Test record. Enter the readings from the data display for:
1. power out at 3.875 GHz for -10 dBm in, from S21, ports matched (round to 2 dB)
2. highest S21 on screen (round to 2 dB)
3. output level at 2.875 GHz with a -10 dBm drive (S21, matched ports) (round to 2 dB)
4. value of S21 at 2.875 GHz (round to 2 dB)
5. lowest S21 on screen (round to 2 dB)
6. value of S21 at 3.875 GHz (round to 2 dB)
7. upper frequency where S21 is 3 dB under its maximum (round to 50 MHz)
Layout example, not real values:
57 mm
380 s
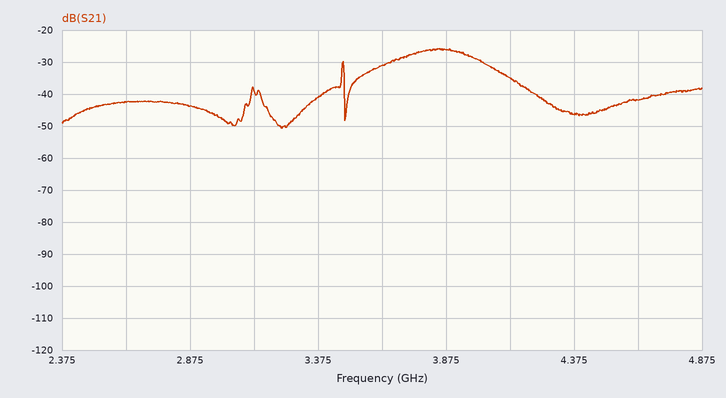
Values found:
-36 dBm
-26 dB
-54 dBm
-44 dB
-50 dB
-26 dB
4.00 GHz
